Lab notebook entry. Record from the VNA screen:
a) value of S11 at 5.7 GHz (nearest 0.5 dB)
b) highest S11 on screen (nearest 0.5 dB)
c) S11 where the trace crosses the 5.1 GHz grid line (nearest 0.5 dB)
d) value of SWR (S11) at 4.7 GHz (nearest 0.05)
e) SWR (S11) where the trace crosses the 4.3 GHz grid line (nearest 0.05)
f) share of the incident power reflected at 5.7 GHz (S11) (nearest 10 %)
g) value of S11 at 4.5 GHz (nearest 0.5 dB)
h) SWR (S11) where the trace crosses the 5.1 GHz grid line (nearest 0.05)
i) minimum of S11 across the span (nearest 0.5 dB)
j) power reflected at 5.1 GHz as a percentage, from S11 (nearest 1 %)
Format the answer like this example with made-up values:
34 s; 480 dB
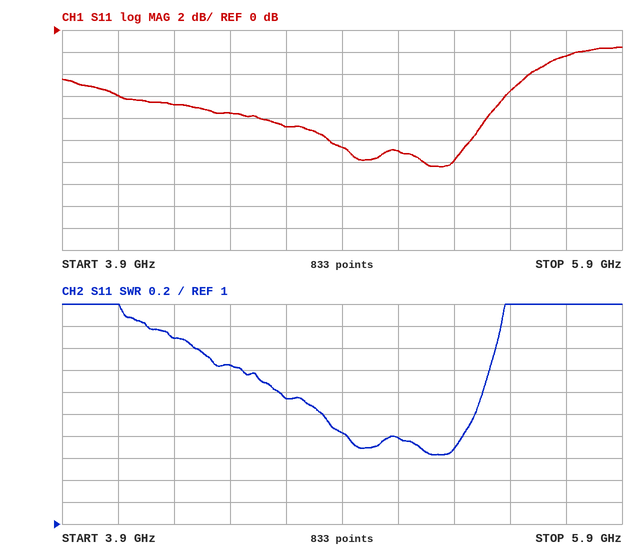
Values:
-2.5 dB; -1.5 dB; -11.0 dB; 2.15; 2.70; 60 %; -7.5 dB; 1.80; -12.5 dB; 8 %
